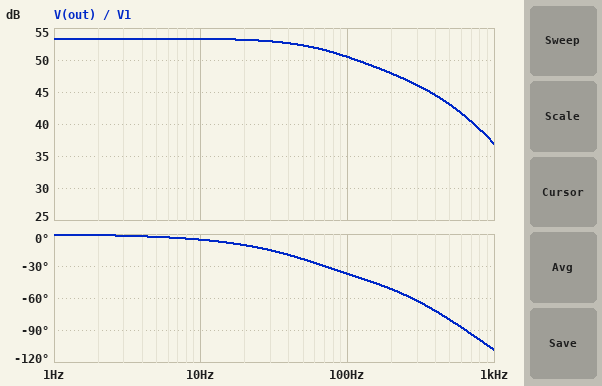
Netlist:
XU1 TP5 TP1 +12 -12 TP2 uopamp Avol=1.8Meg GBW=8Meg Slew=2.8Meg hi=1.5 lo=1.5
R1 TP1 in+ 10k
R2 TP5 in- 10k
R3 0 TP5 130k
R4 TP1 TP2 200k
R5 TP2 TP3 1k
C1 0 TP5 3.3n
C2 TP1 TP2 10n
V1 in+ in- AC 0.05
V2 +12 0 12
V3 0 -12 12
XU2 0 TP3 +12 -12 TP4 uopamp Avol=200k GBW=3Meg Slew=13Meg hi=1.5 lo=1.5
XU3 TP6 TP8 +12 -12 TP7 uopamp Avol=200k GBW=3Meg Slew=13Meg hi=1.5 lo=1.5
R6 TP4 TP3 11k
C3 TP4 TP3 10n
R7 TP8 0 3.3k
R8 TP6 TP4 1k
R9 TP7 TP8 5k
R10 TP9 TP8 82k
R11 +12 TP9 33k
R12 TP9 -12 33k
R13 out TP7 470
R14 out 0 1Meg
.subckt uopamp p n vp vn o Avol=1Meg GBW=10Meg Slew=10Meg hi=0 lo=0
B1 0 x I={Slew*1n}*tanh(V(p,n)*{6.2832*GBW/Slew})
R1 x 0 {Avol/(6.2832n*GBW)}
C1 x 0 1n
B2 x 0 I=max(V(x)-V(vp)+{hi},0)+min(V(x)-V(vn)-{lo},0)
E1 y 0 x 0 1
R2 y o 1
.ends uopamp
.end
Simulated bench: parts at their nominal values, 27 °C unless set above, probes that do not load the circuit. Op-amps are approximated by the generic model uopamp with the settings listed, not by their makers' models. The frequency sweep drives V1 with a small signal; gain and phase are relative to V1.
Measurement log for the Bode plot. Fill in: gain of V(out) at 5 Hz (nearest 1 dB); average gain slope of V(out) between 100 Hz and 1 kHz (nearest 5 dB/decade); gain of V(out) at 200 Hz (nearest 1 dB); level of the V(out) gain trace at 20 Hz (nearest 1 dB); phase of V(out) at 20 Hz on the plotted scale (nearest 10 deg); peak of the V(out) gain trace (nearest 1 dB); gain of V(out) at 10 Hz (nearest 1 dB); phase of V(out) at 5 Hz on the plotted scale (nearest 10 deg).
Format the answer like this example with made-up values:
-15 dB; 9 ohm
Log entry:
53 dB; -15 dB/decade; 48 dB; 53 dB; -10 deg; 53 dB; 53 dB; 0 deg
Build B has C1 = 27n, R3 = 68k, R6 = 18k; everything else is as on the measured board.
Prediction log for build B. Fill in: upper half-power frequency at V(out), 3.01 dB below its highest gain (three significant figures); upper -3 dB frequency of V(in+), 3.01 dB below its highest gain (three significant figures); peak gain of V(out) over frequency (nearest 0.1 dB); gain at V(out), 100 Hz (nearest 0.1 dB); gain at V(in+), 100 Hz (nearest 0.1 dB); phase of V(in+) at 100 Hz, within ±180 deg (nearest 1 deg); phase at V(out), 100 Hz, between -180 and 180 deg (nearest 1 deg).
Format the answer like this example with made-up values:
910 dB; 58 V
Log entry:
80.6 Hz; 89.4 Hz; 55.8 dB; 51.8 dB; 5.7 dB; 120 deg; -57 deg
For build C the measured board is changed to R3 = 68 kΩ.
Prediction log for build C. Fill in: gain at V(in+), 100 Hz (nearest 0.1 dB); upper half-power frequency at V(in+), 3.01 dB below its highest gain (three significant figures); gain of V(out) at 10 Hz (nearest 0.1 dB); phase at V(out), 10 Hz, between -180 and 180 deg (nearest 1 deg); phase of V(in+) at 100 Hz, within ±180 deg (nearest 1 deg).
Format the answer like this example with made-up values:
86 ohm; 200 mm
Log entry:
9.2 dB; 731 Hz; 51.5 dB; -6 deg; 171 deg
